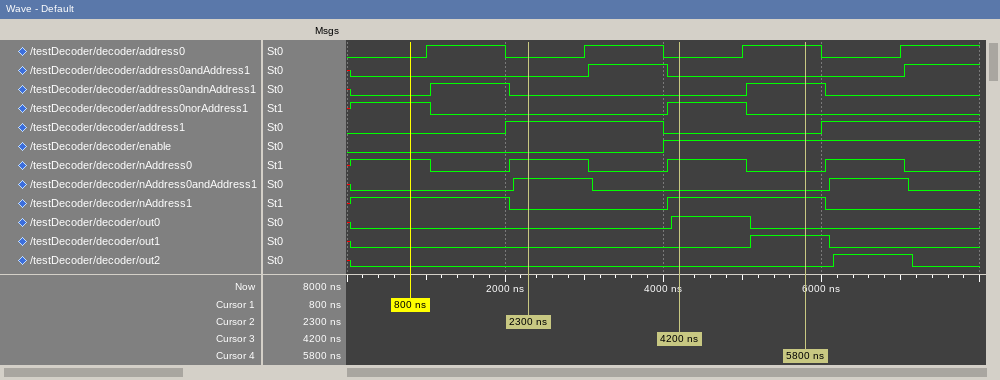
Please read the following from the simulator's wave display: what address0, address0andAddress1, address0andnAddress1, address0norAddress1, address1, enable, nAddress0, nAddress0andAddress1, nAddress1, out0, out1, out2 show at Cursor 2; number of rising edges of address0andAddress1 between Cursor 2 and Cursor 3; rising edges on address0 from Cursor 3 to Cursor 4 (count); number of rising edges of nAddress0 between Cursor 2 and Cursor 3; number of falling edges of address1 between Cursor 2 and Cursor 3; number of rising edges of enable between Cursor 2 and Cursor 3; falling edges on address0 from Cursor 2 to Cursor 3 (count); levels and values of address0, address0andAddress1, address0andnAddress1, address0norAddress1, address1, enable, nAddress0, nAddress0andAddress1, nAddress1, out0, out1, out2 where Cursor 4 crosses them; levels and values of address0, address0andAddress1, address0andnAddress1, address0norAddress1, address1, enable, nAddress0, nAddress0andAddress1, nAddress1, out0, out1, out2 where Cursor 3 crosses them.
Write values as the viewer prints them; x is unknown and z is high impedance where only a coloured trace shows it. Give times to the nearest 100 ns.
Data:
address0=0, address0andAddress1=0, address0andnAddress1=0, address0norAddress1=0, address1=1, enable=0, nAddress0=1, nAddress0andAddress1=1, nAddress1=0, out0=0, out1=0, out2=0
1
1
1
1
1
1
address0=1, address0andAddress1=0, address0andnAddress1=1, address0norAddress1=0, address1=0, enable=1, nAddress0=0, nAddress0andAddress1=0, nAddress1=1, out0=0, out1=1, out2=0
address0=0, address0andAddress1=0, address0andnAddress1=0, address0norAddress1=1, address1=0, enable=1, nAddress0=1, nAddress0andAddress1=0, nAddress1=1, out0=1, out1=0, out2=0
